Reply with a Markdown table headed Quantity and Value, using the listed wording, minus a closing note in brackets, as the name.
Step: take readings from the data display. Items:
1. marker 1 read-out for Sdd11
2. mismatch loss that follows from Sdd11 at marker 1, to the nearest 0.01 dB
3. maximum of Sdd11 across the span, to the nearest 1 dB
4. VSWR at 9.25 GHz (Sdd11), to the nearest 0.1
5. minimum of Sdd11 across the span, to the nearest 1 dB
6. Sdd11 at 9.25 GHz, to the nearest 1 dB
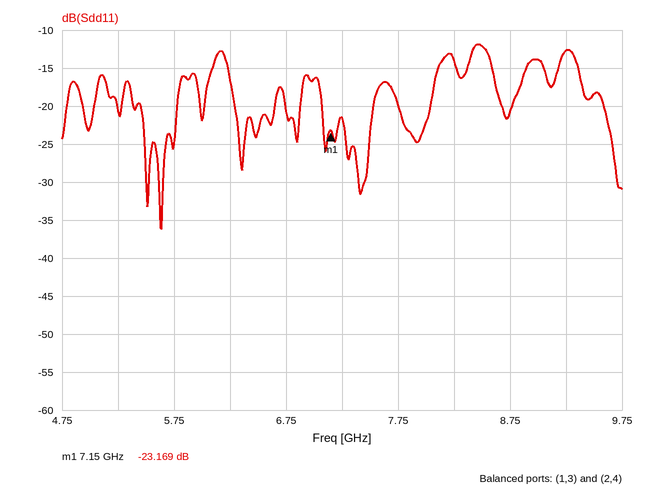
| Quantity | Value |
|---|---|
| marker 1 read-out for Sdd11 | -23.169 dB |
| mismatch loss that follows from Sdd11 at marker 1, to the nearest 0.01 dB | 0.02 dB |
| maximum of Sdd11 across the span, to the nearest 1 dB | -12 dB |
| VSWR at 9.25 GHz (Sdd11), to the nearest 0.1 | 1.6 |
| minimum of Sdd11 across the span, to the nearest 1 dB | -36 dB |
| Sdd11 at 9.25 GHz, to the nearest 1 dB | -13 dB |
